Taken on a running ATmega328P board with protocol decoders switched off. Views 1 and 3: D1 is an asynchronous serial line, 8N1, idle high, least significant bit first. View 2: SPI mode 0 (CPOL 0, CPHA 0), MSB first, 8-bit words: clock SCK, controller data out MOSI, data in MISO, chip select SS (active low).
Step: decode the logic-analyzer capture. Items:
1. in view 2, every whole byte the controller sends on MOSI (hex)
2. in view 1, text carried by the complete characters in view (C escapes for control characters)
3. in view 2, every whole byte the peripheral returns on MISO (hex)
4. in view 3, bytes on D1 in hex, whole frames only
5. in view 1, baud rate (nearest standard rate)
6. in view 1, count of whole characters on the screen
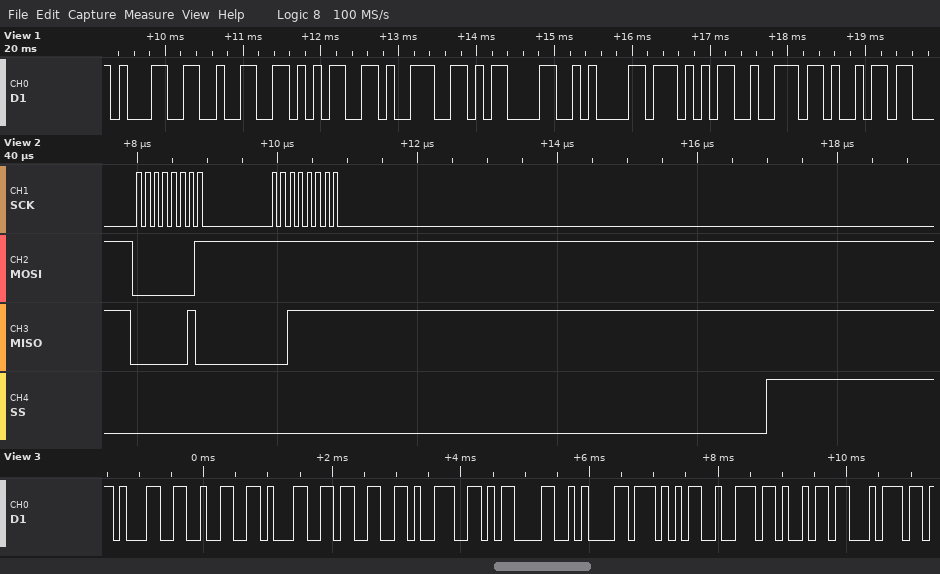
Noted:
01 FF
"1259\r\nWri"
02 3F
31 32 31 33 39 0D 0A 57 72 69 74
9600 baud
9
